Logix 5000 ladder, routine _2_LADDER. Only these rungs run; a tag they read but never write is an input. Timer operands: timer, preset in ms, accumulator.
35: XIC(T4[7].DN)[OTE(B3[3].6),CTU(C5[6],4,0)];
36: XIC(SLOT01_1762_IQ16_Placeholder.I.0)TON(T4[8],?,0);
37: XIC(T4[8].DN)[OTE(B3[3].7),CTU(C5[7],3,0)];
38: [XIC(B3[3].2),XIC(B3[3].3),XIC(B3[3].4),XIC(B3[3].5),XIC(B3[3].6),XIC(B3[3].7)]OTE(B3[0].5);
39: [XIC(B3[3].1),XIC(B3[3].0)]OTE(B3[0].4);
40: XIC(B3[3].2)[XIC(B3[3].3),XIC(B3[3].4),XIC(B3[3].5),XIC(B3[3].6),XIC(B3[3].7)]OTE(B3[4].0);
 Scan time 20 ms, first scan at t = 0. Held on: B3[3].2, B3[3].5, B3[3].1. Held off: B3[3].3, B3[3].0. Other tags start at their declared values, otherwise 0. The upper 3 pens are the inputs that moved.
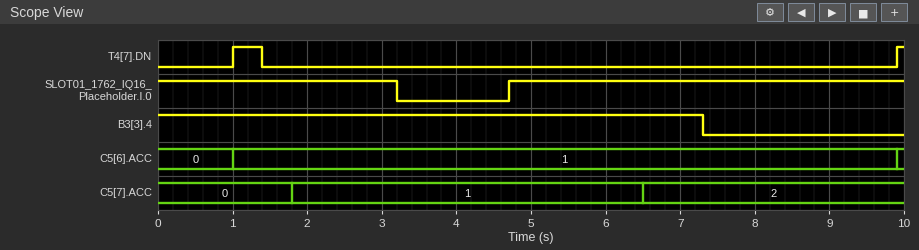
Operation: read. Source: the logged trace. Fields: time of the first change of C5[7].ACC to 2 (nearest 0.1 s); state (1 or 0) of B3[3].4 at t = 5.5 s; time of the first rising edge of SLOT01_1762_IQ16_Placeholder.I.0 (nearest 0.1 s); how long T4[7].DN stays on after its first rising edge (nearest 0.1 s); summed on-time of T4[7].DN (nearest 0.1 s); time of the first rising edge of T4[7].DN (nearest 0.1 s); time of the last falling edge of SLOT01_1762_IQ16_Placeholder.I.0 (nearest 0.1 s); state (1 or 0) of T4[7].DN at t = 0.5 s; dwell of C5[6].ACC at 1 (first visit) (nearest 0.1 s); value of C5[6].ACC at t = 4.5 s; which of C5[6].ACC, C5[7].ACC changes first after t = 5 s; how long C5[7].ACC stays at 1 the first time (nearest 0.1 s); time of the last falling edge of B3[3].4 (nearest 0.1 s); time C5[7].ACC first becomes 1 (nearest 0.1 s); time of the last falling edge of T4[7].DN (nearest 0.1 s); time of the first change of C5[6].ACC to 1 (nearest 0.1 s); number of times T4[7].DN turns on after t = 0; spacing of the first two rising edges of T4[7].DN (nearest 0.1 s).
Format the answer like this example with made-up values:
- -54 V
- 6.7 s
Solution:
- 6.5 s
- 1
- 4.7 s
- 0.4 s
- 0.5 s
- 1.0 s
- 3.2 s
- 0
- 8.9 s
- 1
- C5[7].ACC
- 4.7 s
- 7.3 s
- 1.8 s
- 1.4 s
- 1.0 s
- 2
- 8.9 s
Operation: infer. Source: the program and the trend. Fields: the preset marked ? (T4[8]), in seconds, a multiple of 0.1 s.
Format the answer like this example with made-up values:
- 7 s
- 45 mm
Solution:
- 1.8 s
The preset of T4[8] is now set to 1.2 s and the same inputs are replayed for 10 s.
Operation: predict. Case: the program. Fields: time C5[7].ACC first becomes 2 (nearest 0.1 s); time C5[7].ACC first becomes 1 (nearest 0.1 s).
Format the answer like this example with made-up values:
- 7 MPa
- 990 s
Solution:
- 5.9 s
- 1.2 s
